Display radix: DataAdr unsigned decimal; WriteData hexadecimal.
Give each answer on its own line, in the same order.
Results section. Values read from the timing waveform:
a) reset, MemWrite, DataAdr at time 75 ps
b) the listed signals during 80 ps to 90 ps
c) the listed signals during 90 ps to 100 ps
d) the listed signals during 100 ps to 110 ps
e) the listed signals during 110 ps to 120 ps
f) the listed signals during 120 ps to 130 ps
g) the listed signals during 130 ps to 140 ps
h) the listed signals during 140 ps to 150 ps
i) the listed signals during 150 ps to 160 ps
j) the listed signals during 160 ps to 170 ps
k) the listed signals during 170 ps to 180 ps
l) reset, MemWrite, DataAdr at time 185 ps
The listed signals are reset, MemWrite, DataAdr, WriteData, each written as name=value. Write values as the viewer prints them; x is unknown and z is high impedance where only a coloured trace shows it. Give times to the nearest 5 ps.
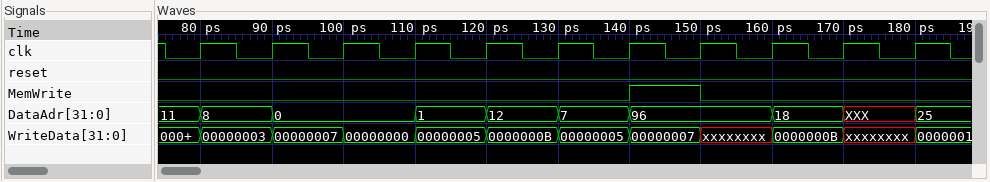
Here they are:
reset=0, MemWrite=0, DataAdr=11
reset=0, MemWrite=0, DataAdr=8, WriteData=00000003
reset=0, MemWrite=0, DataAdr=0, WriteData=00000007
reset=0, MemWrite=0, DataAdr=0, WriteData=00000000
reset=0, MemWrite=0, DataAdr=1, WriteData=00000005
reset=0, MemWrite=0, DataAdr=12, WriteData=0000000B
reset=0, MemWrite=0, DataAdr=7, WriteData=00000005
reset=0, MemWrite=1, DataAdr=96, WriteData=00000007
reset=0, MemWrite=0, DataAdr=96, WriteData=xxxxxxxx
reset=0, MemWrite=0, DataAdr=18, WriteData=0000000B
reset=0, MemWrite=0, DataAdr=XXX, WriteData=xxxxxxxx
reset=0, MemWrite=0, DataAdr=25
